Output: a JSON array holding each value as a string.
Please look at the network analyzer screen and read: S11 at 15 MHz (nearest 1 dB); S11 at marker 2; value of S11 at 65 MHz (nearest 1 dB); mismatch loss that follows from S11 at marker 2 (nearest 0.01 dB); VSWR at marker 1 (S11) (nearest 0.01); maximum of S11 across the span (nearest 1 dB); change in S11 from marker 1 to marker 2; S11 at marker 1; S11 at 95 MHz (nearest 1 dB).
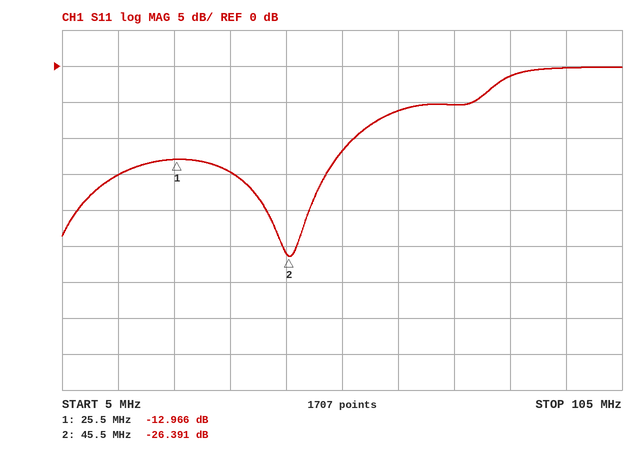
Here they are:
["-15 dB", "-26.391 dB", "-6 dB", "0.01 dB", "1.58", "0 dB", "-13.425 dB", "-12.966 dB", "0 dB"]
